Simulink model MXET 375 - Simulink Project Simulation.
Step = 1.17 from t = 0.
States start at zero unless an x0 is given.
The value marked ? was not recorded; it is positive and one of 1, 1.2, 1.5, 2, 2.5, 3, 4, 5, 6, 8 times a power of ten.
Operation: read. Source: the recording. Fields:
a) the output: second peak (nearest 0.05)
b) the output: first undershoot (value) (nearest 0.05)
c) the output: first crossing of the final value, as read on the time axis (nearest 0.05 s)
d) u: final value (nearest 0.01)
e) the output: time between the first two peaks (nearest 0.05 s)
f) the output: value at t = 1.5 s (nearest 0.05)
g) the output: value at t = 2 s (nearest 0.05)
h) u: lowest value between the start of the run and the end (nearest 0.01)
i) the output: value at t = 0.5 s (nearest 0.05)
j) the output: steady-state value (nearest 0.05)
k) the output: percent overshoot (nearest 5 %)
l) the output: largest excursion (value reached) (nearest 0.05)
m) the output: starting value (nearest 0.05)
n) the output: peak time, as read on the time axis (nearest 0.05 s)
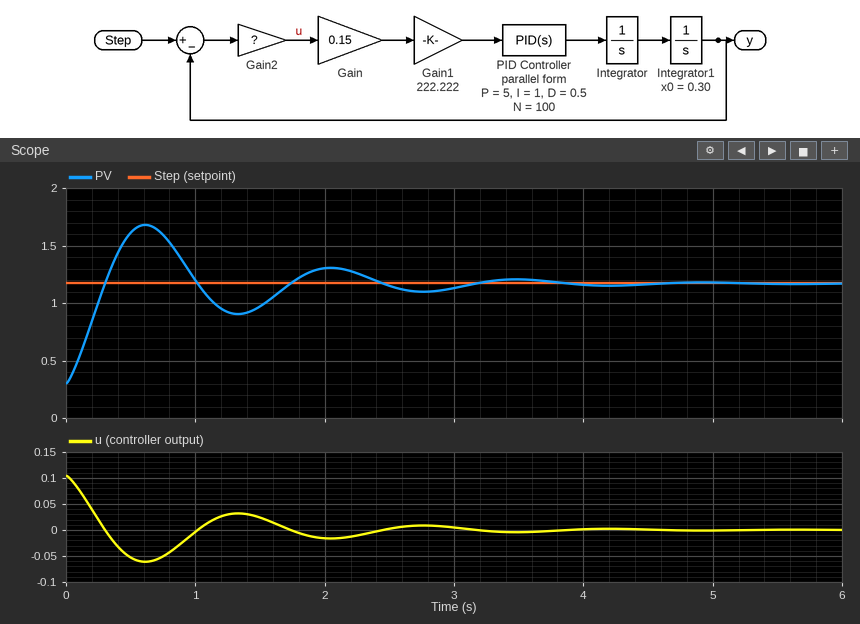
1.30
0.90
0.30 s
0.00
1.45 s
0.95
1.30
-0.06
1.60
1.15
60 %
1.70
0.30
0.60 s
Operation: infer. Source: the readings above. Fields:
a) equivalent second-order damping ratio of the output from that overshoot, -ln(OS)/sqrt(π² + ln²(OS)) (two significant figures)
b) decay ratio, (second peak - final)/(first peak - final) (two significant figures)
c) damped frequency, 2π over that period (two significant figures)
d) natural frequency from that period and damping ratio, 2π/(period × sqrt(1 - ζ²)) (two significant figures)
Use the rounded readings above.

0.16
0.27
4.3 rad/s
4.4 rad/s
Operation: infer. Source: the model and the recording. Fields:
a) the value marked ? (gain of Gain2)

0.12
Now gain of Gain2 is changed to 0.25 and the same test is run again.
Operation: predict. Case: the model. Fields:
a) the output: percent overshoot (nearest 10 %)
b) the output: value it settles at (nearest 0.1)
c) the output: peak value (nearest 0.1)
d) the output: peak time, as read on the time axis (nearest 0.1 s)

50 %
1.2
1.6
0.4 s
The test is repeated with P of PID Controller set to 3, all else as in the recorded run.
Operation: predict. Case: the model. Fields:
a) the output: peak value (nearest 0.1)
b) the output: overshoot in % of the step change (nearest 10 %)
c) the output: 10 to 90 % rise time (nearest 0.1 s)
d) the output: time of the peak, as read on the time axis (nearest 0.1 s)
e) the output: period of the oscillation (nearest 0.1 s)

1.6
50 %
0.3 s
0.8 s
1.9 s
